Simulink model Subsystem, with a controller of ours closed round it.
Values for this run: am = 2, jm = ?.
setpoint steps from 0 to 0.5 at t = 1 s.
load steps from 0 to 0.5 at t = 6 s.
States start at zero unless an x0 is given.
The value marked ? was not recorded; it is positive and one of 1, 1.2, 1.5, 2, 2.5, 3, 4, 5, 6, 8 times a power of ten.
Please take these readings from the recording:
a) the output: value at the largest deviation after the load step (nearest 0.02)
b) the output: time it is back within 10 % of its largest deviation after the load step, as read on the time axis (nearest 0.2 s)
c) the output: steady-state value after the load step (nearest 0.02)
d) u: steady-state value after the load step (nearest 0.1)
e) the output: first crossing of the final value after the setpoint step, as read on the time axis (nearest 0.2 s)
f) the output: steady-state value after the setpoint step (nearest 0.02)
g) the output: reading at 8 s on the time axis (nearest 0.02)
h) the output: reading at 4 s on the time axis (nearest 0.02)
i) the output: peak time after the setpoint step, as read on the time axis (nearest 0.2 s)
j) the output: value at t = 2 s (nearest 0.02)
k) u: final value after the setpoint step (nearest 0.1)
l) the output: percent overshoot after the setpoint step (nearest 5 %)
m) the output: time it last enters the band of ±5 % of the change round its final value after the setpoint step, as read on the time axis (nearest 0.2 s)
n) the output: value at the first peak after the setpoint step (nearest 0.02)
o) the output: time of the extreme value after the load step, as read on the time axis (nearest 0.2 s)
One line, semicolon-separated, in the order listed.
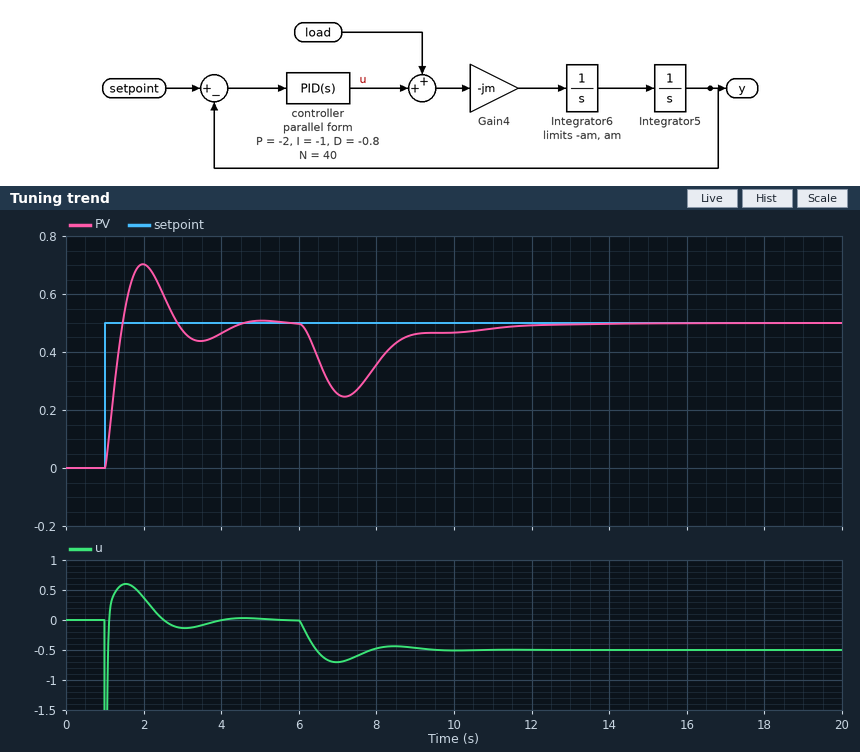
0.24; 10.6 s; 0.50; -0.5; 1.4 s; 0.50; 0.36; 0.46; 2.0 s; 0.70; 0.0; 40 %; 4.2 s; 0.70; 7.2 s
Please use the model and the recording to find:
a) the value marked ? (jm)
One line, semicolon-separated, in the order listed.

3
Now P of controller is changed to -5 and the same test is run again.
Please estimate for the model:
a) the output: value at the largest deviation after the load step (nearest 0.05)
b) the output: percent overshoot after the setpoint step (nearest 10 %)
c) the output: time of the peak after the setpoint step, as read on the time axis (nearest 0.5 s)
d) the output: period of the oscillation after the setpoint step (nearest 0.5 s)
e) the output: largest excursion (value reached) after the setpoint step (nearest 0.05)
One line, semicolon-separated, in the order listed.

0.35; 50 %; 1.5 s; 1.5 s; 0.75
